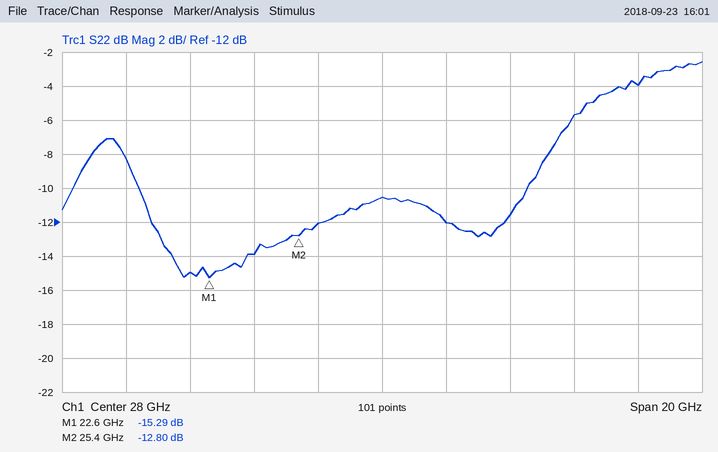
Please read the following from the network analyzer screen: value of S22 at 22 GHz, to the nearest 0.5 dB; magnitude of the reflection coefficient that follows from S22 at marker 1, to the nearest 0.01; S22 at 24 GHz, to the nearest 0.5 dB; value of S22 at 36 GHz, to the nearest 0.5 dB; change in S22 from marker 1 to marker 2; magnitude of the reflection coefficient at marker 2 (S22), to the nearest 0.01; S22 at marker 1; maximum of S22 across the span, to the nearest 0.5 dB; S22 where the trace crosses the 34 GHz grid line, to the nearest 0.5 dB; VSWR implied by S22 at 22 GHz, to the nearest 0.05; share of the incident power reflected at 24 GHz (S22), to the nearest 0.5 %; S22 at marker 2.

-15.0 dB
0.17
-14.0 dB
-4.0 dB
2.49 dB
0.23
-15.29 dB
-2.5 dB
-5.5 dB
1.45
4.0 %
-12.80 dB
